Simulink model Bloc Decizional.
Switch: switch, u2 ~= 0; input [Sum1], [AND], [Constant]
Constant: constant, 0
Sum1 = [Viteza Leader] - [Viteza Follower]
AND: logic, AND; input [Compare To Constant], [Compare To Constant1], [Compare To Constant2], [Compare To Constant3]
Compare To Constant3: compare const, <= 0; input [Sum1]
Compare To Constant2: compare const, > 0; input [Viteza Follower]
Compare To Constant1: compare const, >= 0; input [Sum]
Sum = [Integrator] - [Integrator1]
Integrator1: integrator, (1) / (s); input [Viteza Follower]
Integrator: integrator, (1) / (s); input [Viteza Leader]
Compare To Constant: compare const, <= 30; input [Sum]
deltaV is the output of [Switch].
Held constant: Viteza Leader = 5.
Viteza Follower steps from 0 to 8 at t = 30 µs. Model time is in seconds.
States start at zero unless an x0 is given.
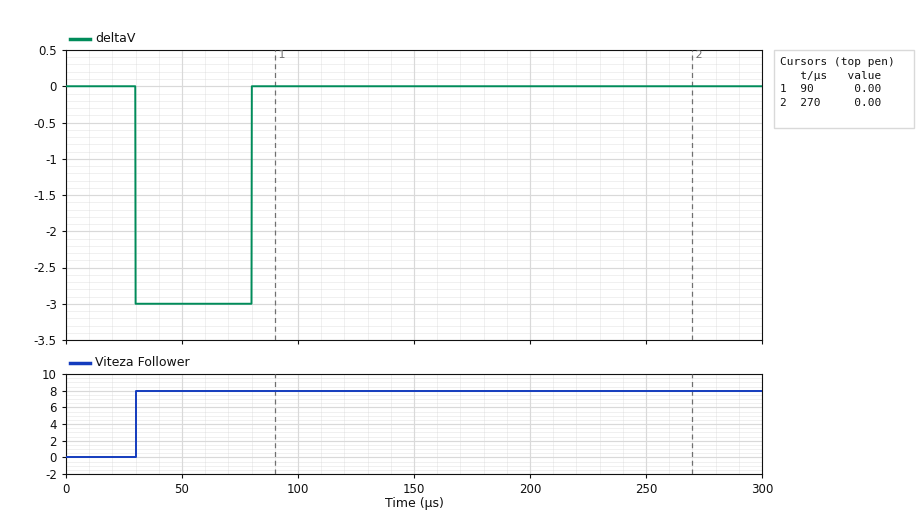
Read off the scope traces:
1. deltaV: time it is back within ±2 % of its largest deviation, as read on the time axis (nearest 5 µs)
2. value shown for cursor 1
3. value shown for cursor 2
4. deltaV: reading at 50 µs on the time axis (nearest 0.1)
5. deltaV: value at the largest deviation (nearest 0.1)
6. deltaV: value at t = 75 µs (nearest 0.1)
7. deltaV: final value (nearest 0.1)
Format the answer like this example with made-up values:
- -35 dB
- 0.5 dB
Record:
- 80 µs
- 0.00
- 0.00
- -3.0
- -3.0
- -3.0
- 0.0
